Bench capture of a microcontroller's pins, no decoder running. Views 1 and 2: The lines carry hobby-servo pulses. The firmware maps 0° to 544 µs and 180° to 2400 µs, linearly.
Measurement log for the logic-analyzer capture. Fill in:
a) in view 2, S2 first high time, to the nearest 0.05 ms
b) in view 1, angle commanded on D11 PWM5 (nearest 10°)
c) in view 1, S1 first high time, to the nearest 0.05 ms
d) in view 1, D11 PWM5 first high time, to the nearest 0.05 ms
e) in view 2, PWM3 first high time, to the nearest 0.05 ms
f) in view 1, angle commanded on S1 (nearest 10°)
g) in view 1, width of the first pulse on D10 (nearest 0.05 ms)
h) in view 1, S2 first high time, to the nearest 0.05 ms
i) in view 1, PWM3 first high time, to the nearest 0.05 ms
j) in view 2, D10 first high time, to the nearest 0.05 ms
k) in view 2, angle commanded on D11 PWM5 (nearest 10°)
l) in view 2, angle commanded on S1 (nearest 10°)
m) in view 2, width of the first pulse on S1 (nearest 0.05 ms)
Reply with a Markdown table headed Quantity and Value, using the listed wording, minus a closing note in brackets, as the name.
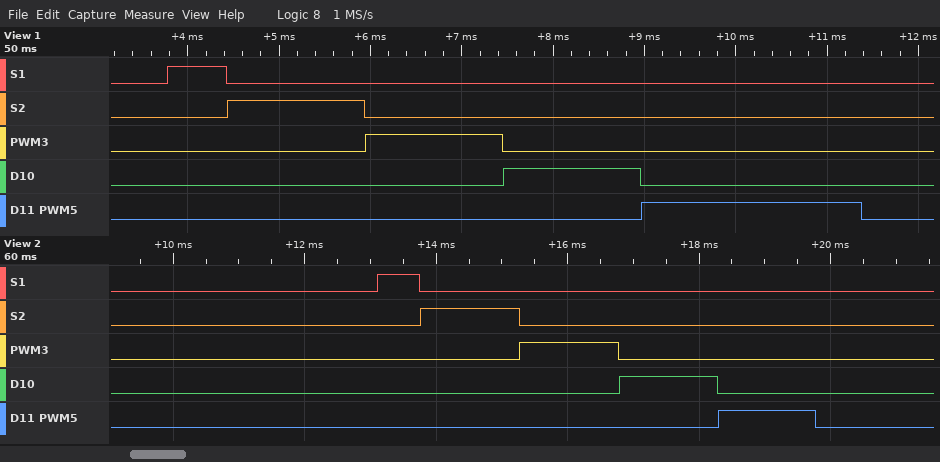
| Quantity | Value |
|---|---|
| in view 2, S2 first high time, to the nearest 0.05 ms | 1.50 ms |
| in view 1, angle commanded on D11 PWM5 | 180° |
| in view 1, S1 first high time, to the nearest 0.05 ms | 0.65 ms |
| in view 1, D11 PWM5 first high time, to the nearest 0.05 ms | 2.40 ms |
| in view 2, PWM3 first high time, to the nearest 0.05 ms | 1.50 ms |
| in view 1, angle commanded on S1 | 10° |
| in view 1, width of the first pulse on D10 | 1.50 ms |
| in view 1, S2 first high time, to the nearest 0.05 ms | 1.50 ms |
| in view 1, PWM3 first high time, to the nearest 0.05 ms | 1.50 ms |
| in view 2, D10 first high time, to the nearest 0.05 ms | 1.50 ms |
| in view 2, angle commanded on D11 PWM5 | 90° |
| in view 2, angle commanded on S1 | 10° |
| in view 2, width of the first pulse on S1 | 0.65 ms |
